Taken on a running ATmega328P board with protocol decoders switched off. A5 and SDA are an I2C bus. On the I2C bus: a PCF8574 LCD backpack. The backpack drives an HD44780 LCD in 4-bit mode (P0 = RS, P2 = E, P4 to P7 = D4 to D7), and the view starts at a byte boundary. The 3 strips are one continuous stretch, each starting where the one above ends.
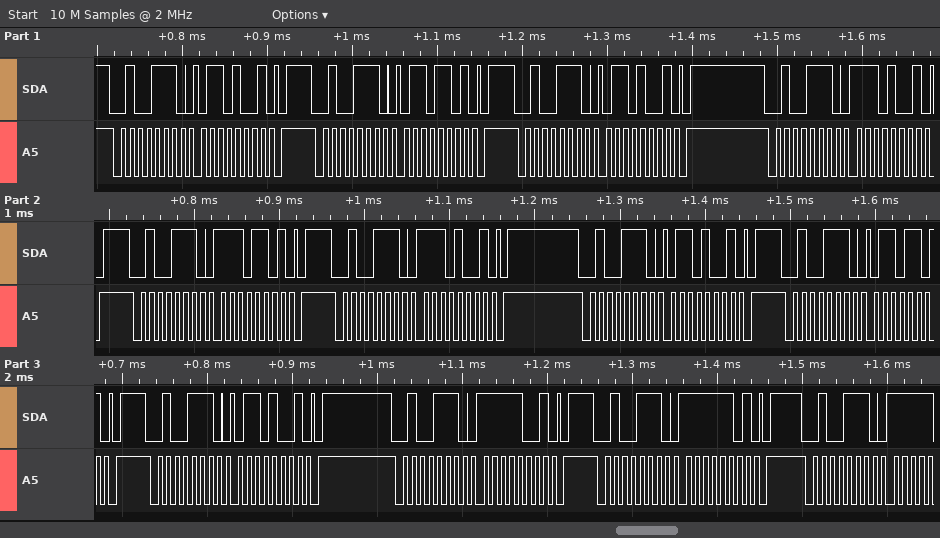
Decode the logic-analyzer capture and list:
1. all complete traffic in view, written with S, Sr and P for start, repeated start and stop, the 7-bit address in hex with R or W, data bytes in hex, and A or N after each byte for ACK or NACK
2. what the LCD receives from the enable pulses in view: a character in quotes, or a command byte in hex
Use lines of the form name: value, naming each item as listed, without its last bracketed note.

all complete traffic in view, written with S, Sr and P for start, repeated start and stop, the 7-bit address in hex with R or W, data bytes in hex, and A or N after each byte for ACK or NACK: S 27W A 69 A P S 27W A 6D A P S 27W A 69 A P S 27W A E9 A P S 27W A ED A P S 27W A E9 A P S 27W A 69 A P S 27W A 6D A P S 27W A 69 A P S 27W A F9 A P S 27W A FD A P S 27W A
what the LCD receives from the enable pulses in view: a character in quotes, or a command byte in hex: 'n'
